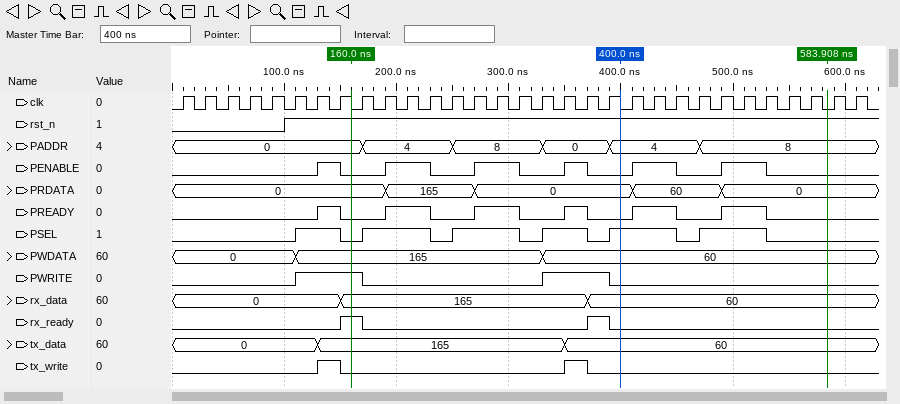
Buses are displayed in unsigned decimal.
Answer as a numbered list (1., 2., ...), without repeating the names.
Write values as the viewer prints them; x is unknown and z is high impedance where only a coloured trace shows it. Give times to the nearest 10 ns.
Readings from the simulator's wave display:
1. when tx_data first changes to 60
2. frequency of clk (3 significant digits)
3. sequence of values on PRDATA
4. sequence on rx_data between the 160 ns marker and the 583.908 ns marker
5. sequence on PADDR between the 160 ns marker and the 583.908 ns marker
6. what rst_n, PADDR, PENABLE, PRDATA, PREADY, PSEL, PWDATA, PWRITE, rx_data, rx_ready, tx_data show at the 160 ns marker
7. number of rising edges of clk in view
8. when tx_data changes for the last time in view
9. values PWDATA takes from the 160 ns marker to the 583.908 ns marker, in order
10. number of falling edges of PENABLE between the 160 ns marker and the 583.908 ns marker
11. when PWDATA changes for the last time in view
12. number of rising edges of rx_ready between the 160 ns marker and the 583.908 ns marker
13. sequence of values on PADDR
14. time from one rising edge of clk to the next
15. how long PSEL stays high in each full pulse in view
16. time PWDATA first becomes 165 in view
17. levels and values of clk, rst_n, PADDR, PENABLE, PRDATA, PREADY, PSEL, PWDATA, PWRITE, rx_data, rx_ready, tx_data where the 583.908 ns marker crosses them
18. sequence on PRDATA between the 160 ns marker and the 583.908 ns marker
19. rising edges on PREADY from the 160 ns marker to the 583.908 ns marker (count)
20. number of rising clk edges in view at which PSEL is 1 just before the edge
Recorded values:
1. 350 ns
2. 50.0 MHz
3. 0, 165, 0, 60, 0
4. 165, 60
5. 0, 4, 8, 0, 4, 8
6. rst_n=1, PADDR=0, PENABLE=0, PRDATA=0, PREADY=0, PSEL=0, PWDATA=165, PWRITE=1, rx_data=165, rx_ready=1, tx_data=165
7. 31
8. 350 ns
9. 165, 60
10. 5
11. 330 ns
12. 1
13. 0, 4, 8, 0, 4, 8
14. 20 ns
15. 40 ns, 60 ns, 60 ns, 40 ns, 60 ns, 60 ns
16. 110 ns
17. clk=0, rst_n=1, PADDR=8, PENABLE=0, PRDATA=0, PREADY=0, PSEL=0, PWDATA=60, PWRITE=0, rx_data=60, rx_ready=0, tx_data=60
18. 0, 165, 0, 60, 0
19. 5
20. 16
